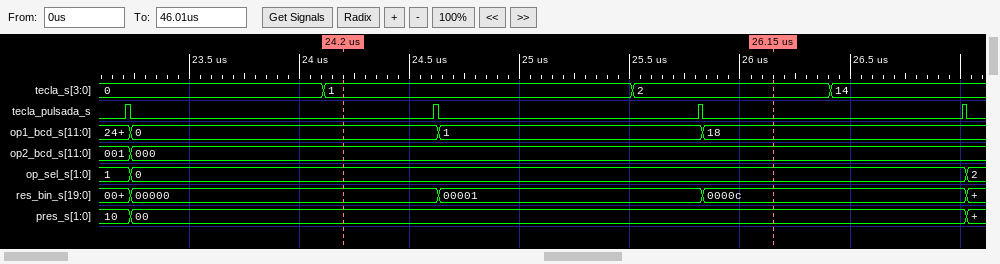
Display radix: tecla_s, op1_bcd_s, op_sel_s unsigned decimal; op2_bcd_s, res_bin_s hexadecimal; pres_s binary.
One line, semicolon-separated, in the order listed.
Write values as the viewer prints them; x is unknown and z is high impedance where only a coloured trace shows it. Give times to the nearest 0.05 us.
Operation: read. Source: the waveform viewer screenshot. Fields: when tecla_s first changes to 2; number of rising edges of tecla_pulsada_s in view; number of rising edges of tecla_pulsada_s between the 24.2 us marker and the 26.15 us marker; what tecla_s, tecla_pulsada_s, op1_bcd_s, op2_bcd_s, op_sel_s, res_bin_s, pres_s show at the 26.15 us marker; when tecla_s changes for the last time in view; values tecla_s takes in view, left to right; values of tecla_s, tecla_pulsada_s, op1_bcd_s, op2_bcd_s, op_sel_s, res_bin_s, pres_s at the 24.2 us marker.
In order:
25.5 us; 4; 2; tecla_s=2, tecla_pulsada_s=0, op1_bcd_s=18, op2_bcd_s=000, op_sel_s=0, res_bin_s=0000c, pres_s=00; 26.4 us; 0, 1, 2, 14; tecla_s=1, tecla_pulsada_s=0, op1_bcd_s=0, op2_bcd_s=000, op_sel_s=0, res_bin_s=00000, pres_s=00
